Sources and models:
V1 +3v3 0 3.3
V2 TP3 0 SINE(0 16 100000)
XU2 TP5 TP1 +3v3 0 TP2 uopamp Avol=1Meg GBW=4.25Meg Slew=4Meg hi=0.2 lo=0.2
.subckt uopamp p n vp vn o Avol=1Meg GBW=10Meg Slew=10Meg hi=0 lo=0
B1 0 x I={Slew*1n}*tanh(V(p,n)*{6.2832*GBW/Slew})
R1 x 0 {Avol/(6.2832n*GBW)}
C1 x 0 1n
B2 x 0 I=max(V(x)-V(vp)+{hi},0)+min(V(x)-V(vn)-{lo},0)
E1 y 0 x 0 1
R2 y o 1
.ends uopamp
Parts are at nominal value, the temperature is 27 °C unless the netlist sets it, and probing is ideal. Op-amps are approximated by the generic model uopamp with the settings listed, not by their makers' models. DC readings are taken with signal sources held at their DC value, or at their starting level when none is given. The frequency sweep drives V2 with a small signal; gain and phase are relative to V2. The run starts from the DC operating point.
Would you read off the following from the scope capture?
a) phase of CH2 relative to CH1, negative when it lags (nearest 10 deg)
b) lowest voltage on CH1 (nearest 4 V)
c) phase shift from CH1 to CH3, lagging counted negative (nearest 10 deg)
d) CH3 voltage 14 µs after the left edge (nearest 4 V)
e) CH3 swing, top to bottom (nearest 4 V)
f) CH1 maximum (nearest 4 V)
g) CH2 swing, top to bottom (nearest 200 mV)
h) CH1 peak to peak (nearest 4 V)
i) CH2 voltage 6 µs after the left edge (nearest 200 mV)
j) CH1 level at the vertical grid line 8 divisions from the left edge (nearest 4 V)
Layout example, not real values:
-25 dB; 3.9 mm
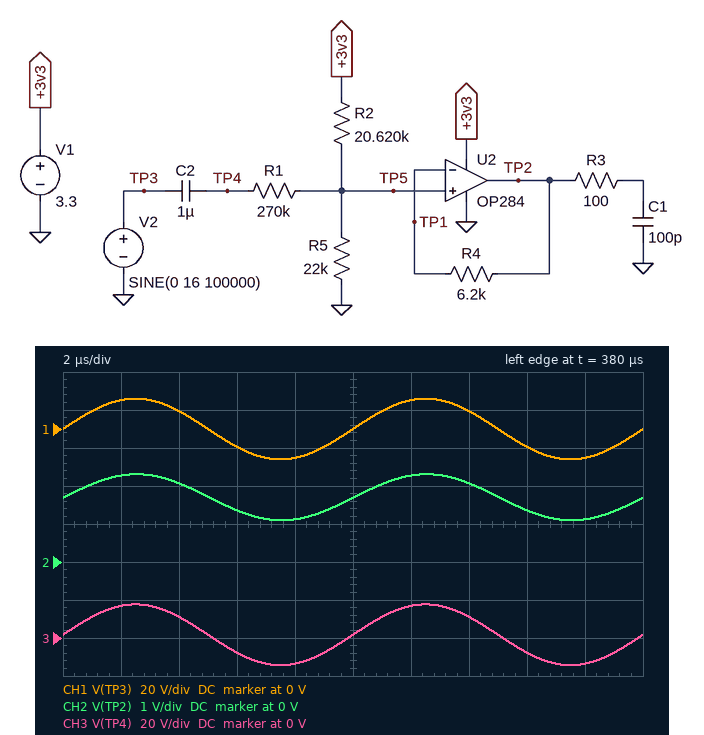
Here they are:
0 deg; -16 V; 0 deg; 12 V; 32 V; 16 V; 1.2 V; 32 V; 1.4 V; -8 V
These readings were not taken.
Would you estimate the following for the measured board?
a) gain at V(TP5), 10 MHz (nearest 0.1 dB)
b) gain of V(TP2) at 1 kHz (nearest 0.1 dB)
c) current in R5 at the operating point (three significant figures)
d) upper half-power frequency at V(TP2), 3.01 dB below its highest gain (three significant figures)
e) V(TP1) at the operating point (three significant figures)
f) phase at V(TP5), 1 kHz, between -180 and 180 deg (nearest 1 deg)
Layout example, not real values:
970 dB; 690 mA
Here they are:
-28.4 dB; -28.4 dB; 77.4 µA; 4.26 MHz; 1.70 V; 0 deg
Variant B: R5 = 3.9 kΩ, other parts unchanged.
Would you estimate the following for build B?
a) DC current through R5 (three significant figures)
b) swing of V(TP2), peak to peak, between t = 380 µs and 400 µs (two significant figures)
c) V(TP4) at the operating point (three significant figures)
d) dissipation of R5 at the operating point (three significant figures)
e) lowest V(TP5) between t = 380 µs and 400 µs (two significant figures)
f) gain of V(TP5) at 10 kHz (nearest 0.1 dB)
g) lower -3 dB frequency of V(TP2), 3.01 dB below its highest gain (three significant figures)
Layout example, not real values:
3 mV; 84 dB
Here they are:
135 µA; 380 mV; 525 mV; 70.6 µW; 330 mV; -38.4 dB; 582 mHz
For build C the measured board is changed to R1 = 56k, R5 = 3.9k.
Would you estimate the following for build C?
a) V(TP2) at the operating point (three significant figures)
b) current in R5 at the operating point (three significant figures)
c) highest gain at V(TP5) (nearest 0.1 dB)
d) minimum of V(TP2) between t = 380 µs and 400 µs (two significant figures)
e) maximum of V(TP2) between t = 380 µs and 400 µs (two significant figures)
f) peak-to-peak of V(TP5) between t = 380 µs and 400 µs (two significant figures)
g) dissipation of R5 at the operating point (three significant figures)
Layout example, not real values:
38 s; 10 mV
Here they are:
525 mV; 135 µA; -25.1 dB; 200 mV; 1.4 V; 1.8 V; 70.6 µW
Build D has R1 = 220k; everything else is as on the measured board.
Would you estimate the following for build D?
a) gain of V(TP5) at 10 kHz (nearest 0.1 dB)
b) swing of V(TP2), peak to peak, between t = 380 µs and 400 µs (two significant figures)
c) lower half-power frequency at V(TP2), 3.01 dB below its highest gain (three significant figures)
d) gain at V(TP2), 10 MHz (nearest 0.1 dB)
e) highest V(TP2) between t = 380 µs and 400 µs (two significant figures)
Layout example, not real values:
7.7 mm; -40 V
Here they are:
-26.7 dB; 1.5 V; 690 mHz; -34.9 dB; 2.4 V
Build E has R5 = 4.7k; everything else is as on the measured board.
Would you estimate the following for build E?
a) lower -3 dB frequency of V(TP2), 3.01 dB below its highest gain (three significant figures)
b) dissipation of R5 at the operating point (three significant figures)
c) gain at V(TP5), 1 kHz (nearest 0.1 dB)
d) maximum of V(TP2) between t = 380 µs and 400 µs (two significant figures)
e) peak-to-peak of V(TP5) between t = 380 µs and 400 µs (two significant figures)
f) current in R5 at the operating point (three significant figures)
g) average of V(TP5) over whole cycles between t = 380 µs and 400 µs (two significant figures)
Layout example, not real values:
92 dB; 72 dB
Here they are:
581 mHz; 79.8 µW; -37.1 dB; 840 mV; 450 mV; 130 µA; 610 mV
